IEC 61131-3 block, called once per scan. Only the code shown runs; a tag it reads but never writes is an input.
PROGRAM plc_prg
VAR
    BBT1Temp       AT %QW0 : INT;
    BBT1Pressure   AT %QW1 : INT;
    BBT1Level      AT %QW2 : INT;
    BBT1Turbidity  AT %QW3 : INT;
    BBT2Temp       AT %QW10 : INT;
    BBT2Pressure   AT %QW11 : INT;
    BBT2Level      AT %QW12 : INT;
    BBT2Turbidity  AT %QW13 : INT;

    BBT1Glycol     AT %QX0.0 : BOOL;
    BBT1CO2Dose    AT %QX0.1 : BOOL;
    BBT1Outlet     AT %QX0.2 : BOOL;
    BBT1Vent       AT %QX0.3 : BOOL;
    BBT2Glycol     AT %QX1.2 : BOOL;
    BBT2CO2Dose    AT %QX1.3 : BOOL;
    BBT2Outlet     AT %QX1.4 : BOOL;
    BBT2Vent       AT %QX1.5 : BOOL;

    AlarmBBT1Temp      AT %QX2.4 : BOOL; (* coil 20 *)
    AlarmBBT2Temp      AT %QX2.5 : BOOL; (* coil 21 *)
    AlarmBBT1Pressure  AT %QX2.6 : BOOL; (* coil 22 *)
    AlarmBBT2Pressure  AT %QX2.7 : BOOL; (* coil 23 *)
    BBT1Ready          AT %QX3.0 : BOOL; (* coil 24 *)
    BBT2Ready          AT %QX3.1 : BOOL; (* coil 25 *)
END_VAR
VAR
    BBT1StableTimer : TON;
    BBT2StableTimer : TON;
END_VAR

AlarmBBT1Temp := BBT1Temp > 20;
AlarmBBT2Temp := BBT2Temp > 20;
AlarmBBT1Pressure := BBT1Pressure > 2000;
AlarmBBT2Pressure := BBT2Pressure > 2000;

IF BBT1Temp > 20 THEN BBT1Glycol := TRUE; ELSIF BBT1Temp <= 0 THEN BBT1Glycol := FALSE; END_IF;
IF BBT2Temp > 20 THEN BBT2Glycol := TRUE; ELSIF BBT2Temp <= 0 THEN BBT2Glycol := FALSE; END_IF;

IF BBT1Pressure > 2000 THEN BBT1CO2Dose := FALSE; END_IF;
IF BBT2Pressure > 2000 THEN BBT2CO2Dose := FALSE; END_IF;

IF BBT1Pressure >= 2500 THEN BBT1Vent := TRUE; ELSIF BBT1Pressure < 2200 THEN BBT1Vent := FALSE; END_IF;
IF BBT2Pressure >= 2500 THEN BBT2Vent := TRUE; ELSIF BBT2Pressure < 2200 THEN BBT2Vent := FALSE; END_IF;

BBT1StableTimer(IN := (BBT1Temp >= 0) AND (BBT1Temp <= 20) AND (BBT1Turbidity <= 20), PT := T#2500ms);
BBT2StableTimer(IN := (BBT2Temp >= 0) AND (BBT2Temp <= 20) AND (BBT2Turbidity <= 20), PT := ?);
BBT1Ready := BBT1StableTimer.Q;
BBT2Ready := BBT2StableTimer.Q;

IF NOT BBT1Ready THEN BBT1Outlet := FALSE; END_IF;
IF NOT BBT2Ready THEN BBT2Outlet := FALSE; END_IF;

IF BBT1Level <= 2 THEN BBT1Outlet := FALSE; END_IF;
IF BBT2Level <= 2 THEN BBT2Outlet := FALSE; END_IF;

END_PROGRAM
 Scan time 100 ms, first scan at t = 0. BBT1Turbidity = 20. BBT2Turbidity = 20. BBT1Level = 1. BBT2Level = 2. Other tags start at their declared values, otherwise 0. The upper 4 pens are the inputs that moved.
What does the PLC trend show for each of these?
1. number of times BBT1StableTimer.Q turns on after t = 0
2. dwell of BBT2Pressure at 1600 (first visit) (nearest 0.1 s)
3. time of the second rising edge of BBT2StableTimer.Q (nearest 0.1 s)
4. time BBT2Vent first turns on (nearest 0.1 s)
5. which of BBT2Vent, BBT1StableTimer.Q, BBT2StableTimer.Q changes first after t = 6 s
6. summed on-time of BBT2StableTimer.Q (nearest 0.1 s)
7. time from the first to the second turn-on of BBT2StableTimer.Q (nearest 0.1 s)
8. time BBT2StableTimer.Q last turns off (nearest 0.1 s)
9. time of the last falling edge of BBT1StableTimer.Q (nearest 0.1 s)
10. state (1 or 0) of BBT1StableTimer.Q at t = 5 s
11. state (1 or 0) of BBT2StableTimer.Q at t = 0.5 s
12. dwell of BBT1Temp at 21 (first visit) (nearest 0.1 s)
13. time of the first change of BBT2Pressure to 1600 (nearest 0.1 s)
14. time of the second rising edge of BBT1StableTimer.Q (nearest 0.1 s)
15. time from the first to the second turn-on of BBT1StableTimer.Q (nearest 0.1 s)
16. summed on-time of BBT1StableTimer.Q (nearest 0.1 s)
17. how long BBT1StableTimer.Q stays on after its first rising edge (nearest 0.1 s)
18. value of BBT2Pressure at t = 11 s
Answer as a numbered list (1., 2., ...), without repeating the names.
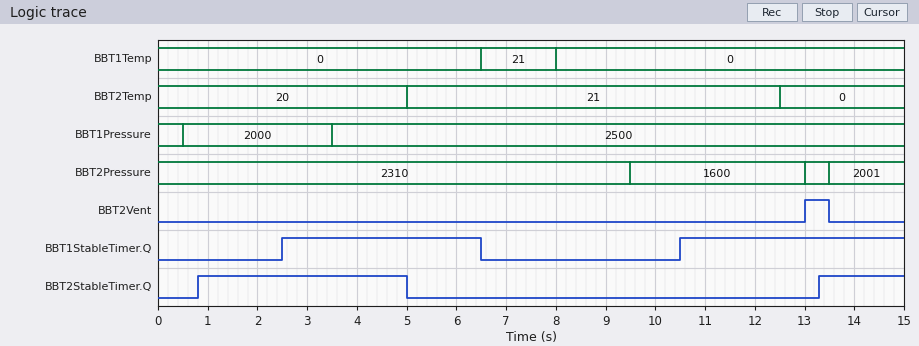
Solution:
1. 2
2. 3.5 s
3. 13.3 s
4. 13.0 s
5. BBT1StableTimer.Q
6. 5.9 s
7. 12.5 s
8. 5.0 s
9. 6.5 s
10. 1
11. 0
12. 1.5 s
13. 9.5 s
14. 10.5 s
15. 8.0 s
16. 8.5 s
17. 4.0 s
18. 1600
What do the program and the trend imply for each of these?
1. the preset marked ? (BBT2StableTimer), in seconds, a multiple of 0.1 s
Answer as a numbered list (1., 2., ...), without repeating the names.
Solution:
1. 0.8 s
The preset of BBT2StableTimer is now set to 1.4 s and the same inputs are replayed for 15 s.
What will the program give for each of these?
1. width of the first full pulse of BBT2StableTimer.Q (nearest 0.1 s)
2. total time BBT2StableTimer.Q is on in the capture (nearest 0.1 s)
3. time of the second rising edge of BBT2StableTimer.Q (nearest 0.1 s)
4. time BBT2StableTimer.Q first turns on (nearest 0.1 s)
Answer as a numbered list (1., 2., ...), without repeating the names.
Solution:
1. 3.6 s
2. 4.7 s
3. 13.9 s
4. 1.4 s
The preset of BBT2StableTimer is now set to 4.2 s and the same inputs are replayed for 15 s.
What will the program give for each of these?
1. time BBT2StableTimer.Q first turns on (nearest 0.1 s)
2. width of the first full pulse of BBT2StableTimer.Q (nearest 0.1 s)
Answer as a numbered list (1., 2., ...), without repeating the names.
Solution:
1. 4.2 s
2. 0.8 s
